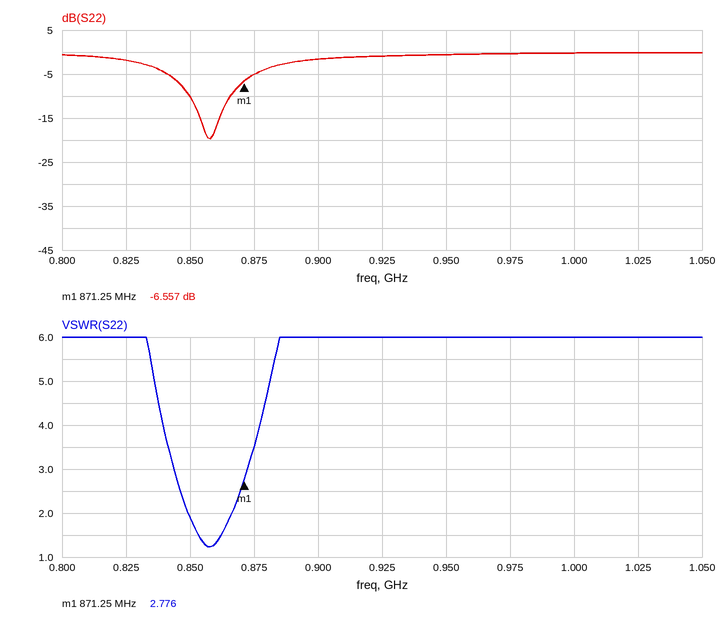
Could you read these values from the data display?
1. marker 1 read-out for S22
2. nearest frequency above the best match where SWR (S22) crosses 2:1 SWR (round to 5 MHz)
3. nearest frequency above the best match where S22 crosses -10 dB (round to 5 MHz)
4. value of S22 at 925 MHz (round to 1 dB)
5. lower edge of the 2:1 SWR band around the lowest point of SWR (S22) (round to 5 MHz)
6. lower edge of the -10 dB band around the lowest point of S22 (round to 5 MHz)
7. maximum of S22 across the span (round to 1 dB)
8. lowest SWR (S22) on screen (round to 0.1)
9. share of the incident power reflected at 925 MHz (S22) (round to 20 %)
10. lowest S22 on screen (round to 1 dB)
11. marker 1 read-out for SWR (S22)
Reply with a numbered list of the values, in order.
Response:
1. -6.557 dB
2. 865 MHz
3. 865 MHz
4. -1 dB
5. 850 MHz
6. 850 MHz
7. 0 dB
8. 1.2
9. 80 %
10. -20 dB
11. 2.776
